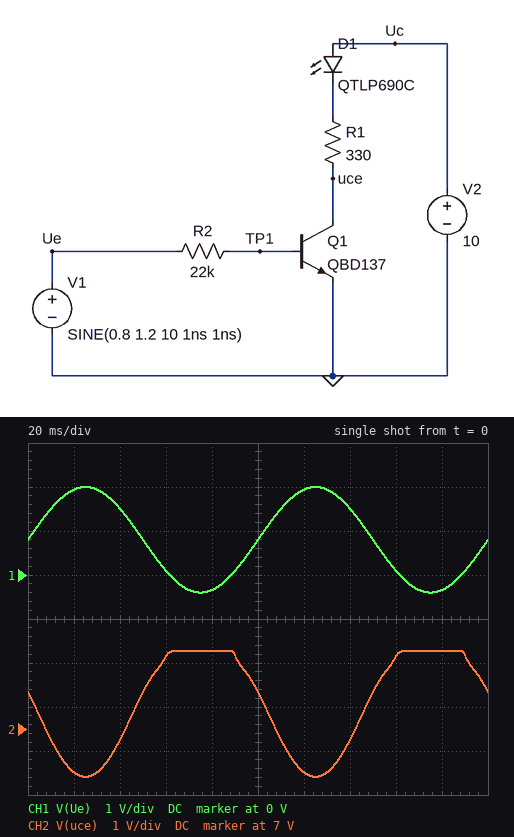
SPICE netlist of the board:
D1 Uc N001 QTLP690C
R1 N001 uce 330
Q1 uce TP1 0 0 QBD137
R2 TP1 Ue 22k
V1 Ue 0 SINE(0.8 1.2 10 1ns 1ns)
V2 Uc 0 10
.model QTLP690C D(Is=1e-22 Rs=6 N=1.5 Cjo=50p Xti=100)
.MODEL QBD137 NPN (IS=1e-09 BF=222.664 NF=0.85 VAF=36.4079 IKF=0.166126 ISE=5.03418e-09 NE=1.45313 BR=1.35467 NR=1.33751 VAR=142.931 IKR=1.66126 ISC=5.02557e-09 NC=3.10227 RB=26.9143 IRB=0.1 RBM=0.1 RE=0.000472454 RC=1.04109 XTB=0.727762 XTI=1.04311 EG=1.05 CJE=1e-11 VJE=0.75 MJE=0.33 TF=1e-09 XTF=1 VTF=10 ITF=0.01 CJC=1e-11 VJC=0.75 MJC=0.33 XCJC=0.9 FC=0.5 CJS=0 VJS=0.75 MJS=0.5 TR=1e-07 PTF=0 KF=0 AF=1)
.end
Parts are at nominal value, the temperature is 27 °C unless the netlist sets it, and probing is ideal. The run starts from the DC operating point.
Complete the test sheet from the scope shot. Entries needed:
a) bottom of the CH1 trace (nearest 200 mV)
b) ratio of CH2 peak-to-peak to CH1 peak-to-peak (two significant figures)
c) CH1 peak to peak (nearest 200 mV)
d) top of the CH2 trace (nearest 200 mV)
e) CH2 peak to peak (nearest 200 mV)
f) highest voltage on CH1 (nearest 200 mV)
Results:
-400 mV
1.2
2.4 V
8.8 V
2.8 V
2.0 V
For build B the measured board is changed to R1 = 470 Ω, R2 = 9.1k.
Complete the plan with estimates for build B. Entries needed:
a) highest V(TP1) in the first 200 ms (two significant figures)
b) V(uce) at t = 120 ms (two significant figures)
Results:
370 mV
270 mV
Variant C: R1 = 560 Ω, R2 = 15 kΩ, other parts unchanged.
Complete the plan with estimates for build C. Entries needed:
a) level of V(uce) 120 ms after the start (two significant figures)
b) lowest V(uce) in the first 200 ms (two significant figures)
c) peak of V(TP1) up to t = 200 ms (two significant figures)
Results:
2.7 V
2.4 V
360 mV
